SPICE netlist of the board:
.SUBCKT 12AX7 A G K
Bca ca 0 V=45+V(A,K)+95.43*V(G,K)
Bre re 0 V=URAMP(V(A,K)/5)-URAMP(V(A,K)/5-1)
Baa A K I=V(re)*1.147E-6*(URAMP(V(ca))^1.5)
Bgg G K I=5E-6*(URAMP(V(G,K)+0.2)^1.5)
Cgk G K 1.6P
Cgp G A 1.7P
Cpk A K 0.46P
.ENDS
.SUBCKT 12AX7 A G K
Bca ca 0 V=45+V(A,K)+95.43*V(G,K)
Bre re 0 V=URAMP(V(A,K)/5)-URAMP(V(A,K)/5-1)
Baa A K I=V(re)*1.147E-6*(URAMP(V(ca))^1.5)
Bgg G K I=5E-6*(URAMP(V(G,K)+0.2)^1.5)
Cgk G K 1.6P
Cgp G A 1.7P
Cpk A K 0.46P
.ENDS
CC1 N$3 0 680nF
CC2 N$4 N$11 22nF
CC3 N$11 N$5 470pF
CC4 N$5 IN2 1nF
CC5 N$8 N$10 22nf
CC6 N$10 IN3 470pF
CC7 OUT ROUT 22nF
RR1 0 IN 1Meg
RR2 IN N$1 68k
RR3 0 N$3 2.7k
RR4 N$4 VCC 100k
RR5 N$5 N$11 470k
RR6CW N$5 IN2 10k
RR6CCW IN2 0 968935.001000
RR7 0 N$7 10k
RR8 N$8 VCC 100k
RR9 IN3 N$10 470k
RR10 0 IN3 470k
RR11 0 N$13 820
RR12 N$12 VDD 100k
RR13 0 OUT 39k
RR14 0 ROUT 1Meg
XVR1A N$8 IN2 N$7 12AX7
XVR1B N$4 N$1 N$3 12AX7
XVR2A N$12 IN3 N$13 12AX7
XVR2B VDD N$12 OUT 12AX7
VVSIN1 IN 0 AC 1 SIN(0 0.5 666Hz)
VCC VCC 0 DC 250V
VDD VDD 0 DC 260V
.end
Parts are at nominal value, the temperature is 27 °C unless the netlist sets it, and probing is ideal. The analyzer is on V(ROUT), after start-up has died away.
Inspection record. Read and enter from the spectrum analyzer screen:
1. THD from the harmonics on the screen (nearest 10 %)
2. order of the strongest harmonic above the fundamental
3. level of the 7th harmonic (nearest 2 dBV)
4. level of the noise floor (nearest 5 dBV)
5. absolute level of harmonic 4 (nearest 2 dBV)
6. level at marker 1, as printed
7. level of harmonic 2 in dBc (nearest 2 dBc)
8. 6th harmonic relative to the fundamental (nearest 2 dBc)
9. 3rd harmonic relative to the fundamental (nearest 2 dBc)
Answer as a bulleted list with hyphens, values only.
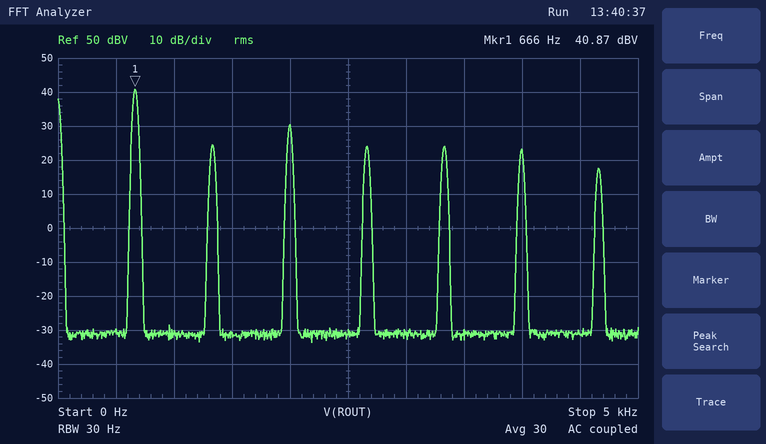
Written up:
- 40 %
- 3
- 18 dBV
- -30 dBV
- 24 dBV
- 40.87 dBV
- -16 dBc
- -18 dBc
- -10 dBc
